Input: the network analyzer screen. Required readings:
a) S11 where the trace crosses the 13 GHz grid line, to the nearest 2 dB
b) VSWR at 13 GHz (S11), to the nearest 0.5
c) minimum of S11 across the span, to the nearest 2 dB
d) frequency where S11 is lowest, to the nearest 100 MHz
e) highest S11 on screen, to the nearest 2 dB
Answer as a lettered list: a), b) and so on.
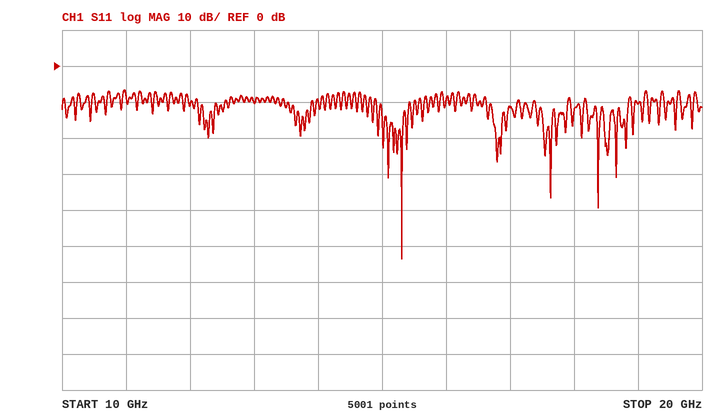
a) -10 dB
b) 2.0
c) -54 dB
d) 15.3 GHz
e) -6 dB
